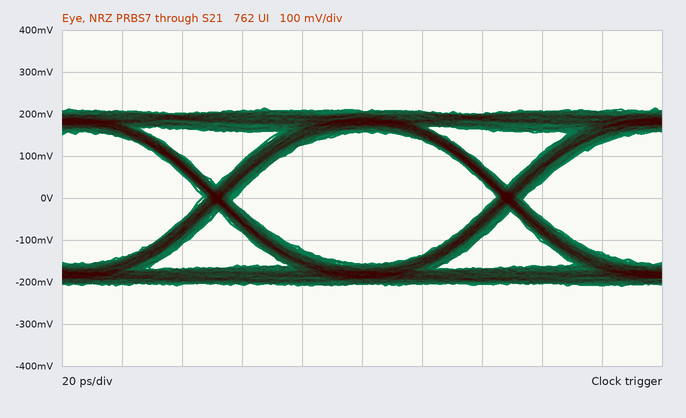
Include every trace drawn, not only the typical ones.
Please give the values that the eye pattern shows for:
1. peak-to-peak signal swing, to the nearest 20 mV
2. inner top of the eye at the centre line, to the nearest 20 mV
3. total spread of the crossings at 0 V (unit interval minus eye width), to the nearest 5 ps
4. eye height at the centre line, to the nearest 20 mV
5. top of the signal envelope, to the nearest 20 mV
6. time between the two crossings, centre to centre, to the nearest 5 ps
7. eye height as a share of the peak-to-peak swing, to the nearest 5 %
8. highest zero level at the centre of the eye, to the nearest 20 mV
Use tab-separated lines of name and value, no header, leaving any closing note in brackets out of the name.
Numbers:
peak-to-peak signal swing, to the nearest 20 mV	420 mV
inner top of the eye at the centre line, to the nearest 20 mV	160 mV
total spread of the crossings at 0 V (unit interval minus eye width), to the nearest 5 ps	10 ps
eye height at the centre line, to the nearest 20 mV	320 mV
top of the signal envelope, to the nearest 20 mV	220 mV
time between the two crossings, centre to centre, to the nearest 5 ps	95 ps
eye height as a share of the peak-to-peak swing, to the nearest 5 %	75 %
highest zero level at the centre of the eye, to the nearest 20 mV	-160 mV
